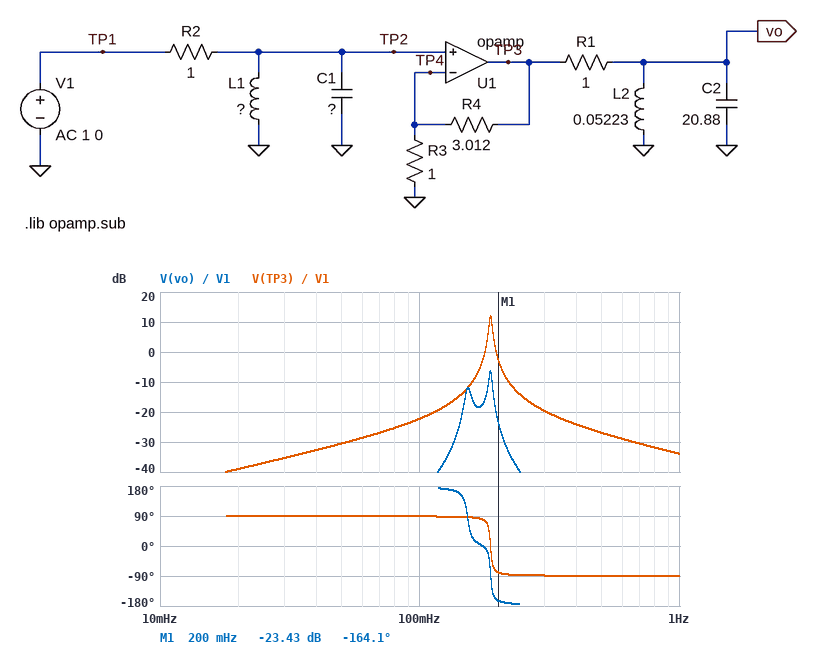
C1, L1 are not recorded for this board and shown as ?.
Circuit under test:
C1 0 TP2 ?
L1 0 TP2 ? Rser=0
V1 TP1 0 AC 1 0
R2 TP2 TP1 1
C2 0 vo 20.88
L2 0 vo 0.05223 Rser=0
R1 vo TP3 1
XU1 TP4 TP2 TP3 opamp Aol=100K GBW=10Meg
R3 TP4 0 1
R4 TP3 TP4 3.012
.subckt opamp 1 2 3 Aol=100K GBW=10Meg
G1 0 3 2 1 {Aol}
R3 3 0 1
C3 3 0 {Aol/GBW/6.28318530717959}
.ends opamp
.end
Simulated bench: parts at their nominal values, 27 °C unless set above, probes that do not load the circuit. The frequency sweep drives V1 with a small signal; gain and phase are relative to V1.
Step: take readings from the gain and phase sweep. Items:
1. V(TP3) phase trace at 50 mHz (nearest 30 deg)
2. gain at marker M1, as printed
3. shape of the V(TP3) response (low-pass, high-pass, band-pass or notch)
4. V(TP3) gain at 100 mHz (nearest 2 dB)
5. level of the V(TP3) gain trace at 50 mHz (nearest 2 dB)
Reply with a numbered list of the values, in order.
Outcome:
1. 90 deg
2. -23.43 dB
3. band-pass
4. -22 dB
5. -30 dB
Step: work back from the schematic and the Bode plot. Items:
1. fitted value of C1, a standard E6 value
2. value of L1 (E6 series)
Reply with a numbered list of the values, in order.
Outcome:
1. 33 F
2. 22 mH
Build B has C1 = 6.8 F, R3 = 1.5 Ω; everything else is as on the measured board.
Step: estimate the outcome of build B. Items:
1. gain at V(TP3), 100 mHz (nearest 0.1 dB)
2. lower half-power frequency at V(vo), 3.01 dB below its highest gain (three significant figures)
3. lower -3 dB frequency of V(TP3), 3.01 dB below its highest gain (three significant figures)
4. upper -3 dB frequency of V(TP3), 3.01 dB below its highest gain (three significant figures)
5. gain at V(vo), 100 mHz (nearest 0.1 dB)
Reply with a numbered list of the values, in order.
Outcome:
1. -27.1 dB
2. 149 mHz
3. 400 mHz
4. 423 mHz
5. -51.9 dB
